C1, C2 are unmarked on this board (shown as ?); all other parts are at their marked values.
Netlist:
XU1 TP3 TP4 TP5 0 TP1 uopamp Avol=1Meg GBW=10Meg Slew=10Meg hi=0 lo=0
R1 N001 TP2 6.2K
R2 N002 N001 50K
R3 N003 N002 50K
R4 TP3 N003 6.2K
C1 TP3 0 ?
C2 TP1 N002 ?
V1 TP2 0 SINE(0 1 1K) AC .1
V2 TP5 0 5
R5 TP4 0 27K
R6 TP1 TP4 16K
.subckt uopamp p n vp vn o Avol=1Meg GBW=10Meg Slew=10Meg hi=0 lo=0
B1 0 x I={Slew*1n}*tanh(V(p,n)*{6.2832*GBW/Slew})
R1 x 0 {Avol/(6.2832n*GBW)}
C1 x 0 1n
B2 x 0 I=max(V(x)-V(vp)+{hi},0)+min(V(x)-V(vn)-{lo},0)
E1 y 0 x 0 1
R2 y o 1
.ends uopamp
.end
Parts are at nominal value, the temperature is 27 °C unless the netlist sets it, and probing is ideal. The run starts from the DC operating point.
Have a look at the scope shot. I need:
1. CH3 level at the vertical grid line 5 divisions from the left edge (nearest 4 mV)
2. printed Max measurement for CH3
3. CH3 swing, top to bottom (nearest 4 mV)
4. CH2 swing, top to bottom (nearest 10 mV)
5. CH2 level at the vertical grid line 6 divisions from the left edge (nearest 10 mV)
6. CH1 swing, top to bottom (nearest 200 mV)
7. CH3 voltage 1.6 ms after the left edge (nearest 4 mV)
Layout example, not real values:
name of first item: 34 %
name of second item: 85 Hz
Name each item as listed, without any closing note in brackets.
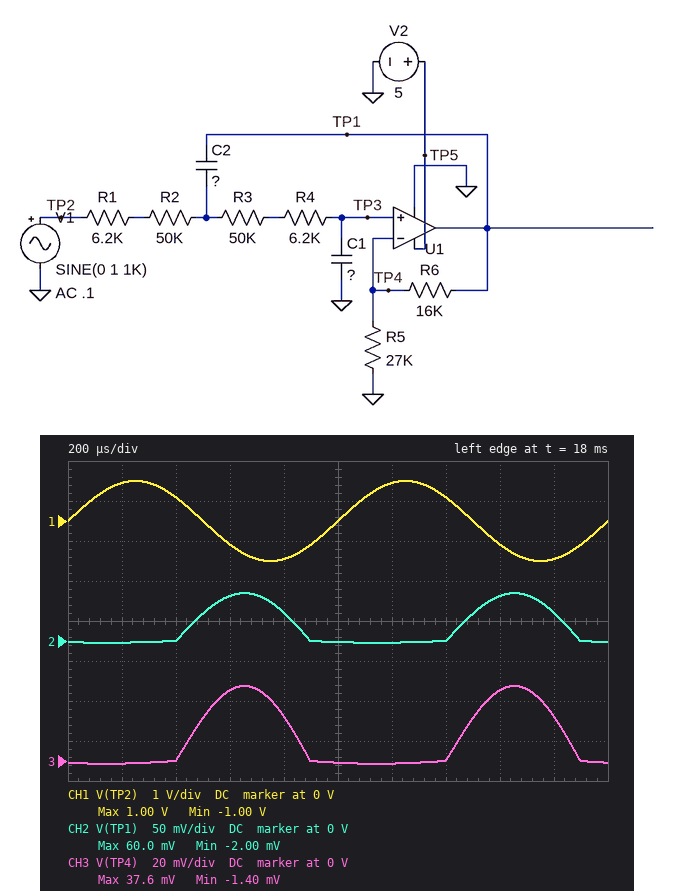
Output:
CH3 level at the vertical grid line 5 divisions from the left edge: 0 V
printed Max measurement for CH3: 37.6 mV
CH3 swing, top to bottom: 40 mV
CH2 swing, top to bottom: 60 mV
CH2 level at the vertical grid line 6 divisions from the left edge: 0 V
CH1 swing, top to bottom: 2.0 V
CH3 voltage 1.6 ms after the left edge: 36 mV
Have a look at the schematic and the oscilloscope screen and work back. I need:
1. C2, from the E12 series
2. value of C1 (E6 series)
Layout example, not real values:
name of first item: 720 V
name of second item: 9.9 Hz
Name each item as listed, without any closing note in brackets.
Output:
C2, from the E12 series: 8.2 nF
value of C1: 22 nF
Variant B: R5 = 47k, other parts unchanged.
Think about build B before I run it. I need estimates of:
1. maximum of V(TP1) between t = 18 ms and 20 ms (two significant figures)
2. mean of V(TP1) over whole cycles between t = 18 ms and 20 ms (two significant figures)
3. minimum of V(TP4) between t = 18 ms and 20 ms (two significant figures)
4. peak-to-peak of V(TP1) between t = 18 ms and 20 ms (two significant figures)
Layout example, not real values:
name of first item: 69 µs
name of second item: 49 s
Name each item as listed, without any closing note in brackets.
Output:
maximum of V(TP1) between t = 18 ms and 20 ms: 50 mV
mean of V(TP1) over whole cycles between t = 18 ms and 20 ms: 15 mV
minimum of V(TP4) between t = 18 ms and 20 ms: -1.6 mV
peak-to-peak of V(TP1) between t = 18 ms and 20 ms: 52 mV
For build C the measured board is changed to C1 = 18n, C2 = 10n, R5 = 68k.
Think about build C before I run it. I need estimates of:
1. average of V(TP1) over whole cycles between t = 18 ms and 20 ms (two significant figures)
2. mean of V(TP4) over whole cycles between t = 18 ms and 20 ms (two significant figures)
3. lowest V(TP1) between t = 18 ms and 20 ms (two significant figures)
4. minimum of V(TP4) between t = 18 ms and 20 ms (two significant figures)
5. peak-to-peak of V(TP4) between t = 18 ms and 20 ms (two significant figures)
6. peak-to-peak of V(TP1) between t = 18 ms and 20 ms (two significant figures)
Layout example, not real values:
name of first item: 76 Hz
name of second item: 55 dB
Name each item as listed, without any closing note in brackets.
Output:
average of V(TP1) over whole cycles between t = 18 ms and 20 ms: 15 mV
mean of V(TP4) over whole cycles between t = 18 ms and 20 ms: 12 mV
lowest V(TP1) between t = 18 ms and 20 ms: -2.3 mV
minimum of V(TP4) between t = 18 ms and 20 ms: -1.8 mV
peak-to-peak of V(TP4) between t = 18 ms and 20 ms: 41 mV
peak-to-peak of V(TP1) between t = 18 ms and 20 ms: 51 mV
